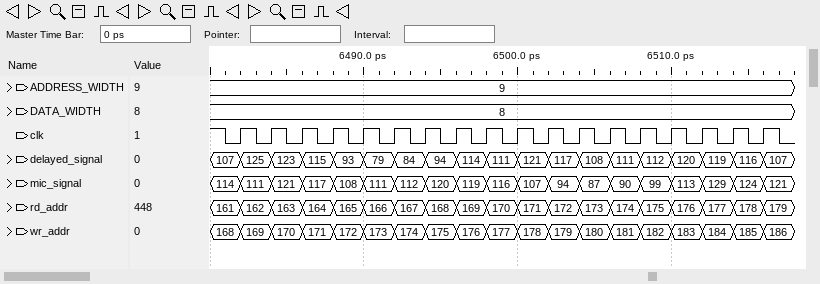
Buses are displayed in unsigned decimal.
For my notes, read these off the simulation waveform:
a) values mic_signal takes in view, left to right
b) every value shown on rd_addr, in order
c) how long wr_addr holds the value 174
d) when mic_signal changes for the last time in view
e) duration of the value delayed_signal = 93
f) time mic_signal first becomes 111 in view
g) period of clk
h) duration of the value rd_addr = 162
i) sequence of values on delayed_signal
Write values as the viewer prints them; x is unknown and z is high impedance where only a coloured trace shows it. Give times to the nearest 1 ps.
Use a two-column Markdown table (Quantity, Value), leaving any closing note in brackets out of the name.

| Quantity | Value |
|---|---|
| values mic_signal takes in view, left to right | 114, 111, 121, 117, 108, 111, 112, 120, 119, 116, 107, 94, 87, 90, 99, 113, 129, 124, 121 |
| every value shown on rd_addr, in order | 161, 162, 163, 164, 165, 166, 167, 168, 169, 170, 171, 172, 173, 174, 175, 176, 177, 178, 179 |
| how long wr_addr holds the value 174 | 2 ps |
| when mic_signal changes for the last time in view | 6516 ps |
| duration of the value delayed_signal = 93 | 2 ps |
| time mic_signal first becomes 111 in view | 6482 ps |
| period of clk | 2 ps |
| duration of the value rd_addr = 162 | 2 ps |
| sequence of values on delayed_signal | 107, 125, 123, 115, 93, 79, 84, 94, 114, 111, 121, 117, 108, 111, 112, 120, 119, 116, 107 |
